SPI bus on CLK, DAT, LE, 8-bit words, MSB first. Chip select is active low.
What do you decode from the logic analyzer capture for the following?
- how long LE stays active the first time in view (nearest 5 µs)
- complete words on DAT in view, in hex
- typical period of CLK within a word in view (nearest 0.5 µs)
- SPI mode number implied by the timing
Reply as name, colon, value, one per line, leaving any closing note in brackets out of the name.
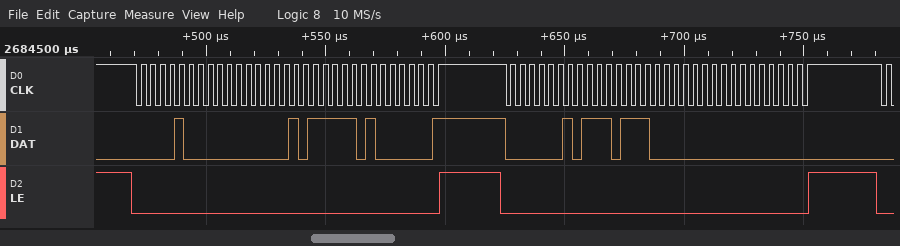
how long LE stays active the first time in view: 130 µs
complete words on DAT in view, in hex: 08, 00, BE, 81, 02, EE, 00, 00
typical period of CLK within a word in view: 4 µs
SPI mode number implied by the timing: 3
